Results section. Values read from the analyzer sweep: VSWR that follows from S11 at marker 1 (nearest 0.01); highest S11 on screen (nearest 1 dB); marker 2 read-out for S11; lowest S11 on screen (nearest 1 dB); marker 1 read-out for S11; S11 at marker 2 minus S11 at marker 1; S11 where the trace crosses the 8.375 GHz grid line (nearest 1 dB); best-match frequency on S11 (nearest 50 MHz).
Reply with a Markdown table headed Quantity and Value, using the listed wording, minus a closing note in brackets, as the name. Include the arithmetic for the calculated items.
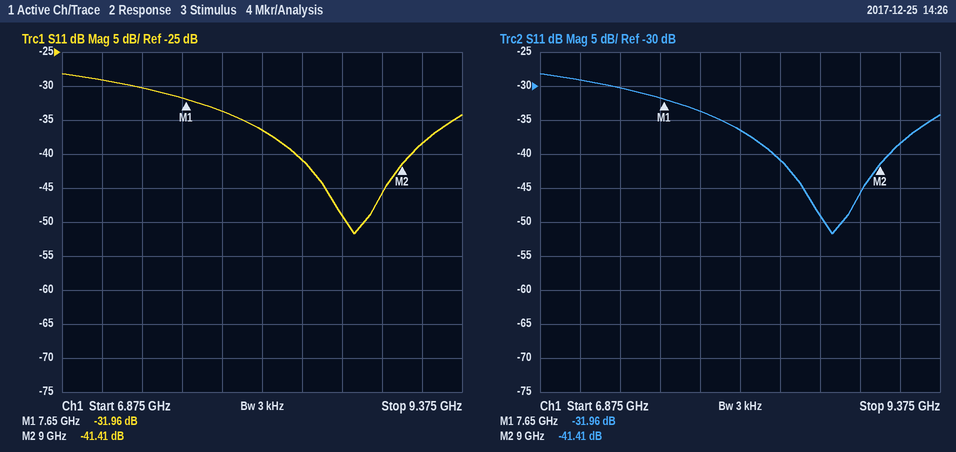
| Quantity | Value |
|---|---|
| VSWR that follows from S11 at marker 1 | (1 + 0.0252)/(1 − 0.0252) ≈ 1.05 |
| highest S11 on screen | -28 dB |
| marker 2 read-out for S11 | -41.41 dB |
| lowest S11 on screen | -52 dB |
| marker 1 read-out for S11 | -31.96 dB |
| S11 at marker 2 minus S11 at marker 1 | -41.41 − (-31.96) = -9.45 dB |
| S11 where the trace crosses the 8.375 GHz grid line | -41 dB |
| best-match frequency on S11 | 8.70 GHz |
